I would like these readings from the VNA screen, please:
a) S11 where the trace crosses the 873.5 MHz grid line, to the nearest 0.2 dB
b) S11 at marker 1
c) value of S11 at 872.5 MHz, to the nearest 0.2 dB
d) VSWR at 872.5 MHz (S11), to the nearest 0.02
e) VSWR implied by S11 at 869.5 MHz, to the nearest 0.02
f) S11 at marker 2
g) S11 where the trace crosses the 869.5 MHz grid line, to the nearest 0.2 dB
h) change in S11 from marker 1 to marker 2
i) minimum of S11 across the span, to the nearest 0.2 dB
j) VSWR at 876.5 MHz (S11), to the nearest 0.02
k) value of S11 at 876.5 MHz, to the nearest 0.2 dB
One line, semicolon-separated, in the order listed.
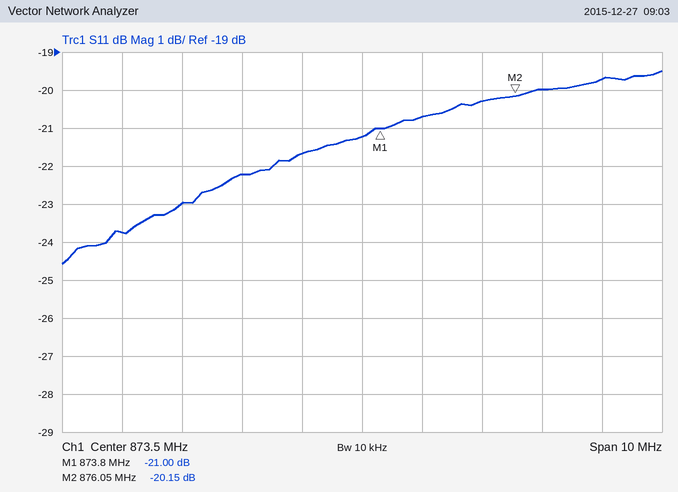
-21.2 dB; -21.00 dB; -21.6 dB; 1.18; 1.14; -20.15 dB; -23.8 dB; 0.85 dB; -24.6 dB; 1.22; -20.0 dB
